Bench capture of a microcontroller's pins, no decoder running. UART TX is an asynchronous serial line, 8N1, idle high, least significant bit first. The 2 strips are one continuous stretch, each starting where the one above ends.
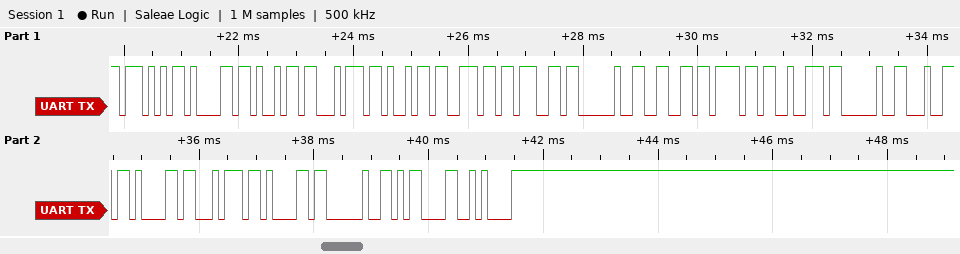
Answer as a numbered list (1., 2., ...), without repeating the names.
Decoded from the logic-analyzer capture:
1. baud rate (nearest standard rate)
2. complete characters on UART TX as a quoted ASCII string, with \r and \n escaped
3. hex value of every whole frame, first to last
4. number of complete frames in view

1. 9600 baud
2. "Waiting for data \r\n"
3. 0x57 0x61 0x69 0x74 0x69 0x6E 0x67 0x20 0x66 0x6F 0x72 0x20 0x64 0x61 0x74 0x61 0x20 0x0D 0x0A
4. 19
